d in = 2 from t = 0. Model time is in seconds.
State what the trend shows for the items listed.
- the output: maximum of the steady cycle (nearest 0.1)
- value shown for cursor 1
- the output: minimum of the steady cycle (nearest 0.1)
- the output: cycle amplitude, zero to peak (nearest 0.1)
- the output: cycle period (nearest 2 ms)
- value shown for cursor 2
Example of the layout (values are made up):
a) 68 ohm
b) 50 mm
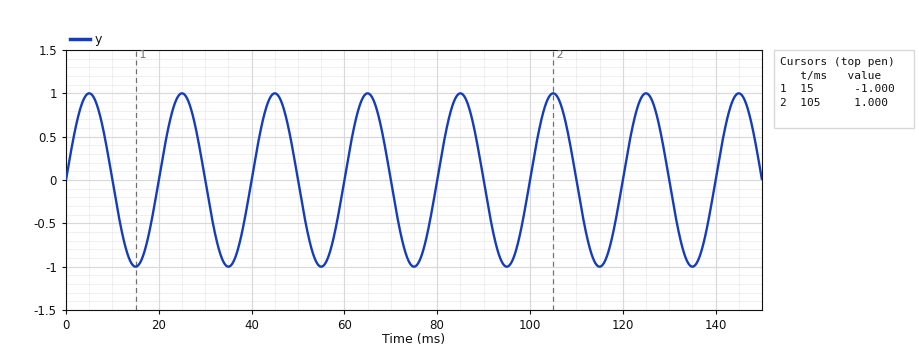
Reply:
a) 1.0
b) -1.000
c) -1.0
d) 1.0
e) 20 ms
f) 1.000
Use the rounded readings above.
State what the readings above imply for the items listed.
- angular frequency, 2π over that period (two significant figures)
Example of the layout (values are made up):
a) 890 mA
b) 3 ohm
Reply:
a) 0.31 rad/ms
